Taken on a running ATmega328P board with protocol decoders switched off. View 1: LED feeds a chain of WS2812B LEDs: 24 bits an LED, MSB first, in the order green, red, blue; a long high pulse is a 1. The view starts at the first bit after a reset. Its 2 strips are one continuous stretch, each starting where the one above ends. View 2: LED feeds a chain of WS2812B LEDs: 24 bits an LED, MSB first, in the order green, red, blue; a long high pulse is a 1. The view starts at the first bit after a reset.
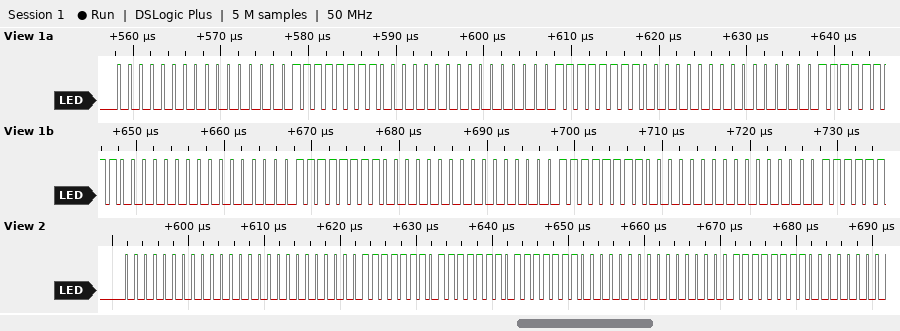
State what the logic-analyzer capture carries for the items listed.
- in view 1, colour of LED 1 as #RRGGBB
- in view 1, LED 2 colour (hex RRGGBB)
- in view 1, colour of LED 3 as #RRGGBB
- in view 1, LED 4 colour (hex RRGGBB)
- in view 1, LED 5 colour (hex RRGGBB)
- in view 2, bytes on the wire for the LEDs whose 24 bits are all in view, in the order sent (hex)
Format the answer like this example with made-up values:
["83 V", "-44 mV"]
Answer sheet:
["#0000FF", "#0000FF", "#0000FF", "#0000FF", "#0000FF", "00 00 00 7F 7F 7F 00 00 FF"]
